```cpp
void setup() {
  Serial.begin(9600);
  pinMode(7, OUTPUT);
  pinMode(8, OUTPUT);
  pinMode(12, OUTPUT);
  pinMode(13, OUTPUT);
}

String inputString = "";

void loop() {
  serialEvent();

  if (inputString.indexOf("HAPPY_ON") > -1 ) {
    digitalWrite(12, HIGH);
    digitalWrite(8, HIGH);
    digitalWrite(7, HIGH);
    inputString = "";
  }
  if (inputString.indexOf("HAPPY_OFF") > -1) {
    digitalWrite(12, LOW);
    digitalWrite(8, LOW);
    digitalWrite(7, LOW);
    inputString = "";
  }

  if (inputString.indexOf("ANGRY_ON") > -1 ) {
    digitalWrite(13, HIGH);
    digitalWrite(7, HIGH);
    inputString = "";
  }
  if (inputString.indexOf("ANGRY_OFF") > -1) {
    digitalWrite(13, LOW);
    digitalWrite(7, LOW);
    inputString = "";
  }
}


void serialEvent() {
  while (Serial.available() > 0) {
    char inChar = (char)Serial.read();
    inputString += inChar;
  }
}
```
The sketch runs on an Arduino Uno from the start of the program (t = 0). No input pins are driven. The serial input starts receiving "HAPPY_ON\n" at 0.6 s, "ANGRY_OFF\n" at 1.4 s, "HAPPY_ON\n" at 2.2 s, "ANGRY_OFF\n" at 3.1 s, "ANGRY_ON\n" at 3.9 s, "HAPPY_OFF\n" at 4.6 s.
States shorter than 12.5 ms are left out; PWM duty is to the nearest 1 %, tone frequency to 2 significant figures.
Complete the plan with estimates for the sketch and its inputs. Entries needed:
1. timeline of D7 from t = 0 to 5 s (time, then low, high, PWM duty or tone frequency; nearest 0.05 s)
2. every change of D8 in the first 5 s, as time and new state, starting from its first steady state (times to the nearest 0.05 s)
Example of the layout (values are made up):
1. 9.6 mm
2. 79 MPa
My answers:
1. 0 s low; 0.6 s high; 1.4 s low; 2.2 s high; 3.1 s low; 3.9 s high; 4.6 s low
2. 0 s low; 0.6 s high; 4.6 s low
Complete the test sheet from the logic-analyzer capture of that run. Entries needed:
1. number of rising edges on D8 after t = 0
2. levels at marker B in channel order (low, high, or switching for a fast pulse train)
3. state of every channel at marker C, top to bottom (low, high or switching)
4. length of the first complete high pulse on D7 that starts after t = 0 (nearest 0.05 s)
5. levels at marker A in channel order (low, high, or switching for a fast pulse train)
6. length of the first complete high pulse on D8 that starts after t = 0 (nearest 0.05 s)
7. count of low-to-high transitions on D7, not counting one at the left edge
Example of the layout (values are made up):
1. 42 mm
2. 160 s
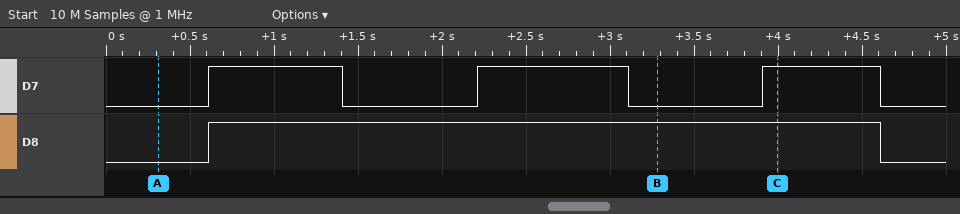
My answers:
1. 1
2. D7 low, D8 high
3. D7 high, D8 high
4. 0.80 s
5. D7 low, D8 low
6. 4.00 s
7. 3
